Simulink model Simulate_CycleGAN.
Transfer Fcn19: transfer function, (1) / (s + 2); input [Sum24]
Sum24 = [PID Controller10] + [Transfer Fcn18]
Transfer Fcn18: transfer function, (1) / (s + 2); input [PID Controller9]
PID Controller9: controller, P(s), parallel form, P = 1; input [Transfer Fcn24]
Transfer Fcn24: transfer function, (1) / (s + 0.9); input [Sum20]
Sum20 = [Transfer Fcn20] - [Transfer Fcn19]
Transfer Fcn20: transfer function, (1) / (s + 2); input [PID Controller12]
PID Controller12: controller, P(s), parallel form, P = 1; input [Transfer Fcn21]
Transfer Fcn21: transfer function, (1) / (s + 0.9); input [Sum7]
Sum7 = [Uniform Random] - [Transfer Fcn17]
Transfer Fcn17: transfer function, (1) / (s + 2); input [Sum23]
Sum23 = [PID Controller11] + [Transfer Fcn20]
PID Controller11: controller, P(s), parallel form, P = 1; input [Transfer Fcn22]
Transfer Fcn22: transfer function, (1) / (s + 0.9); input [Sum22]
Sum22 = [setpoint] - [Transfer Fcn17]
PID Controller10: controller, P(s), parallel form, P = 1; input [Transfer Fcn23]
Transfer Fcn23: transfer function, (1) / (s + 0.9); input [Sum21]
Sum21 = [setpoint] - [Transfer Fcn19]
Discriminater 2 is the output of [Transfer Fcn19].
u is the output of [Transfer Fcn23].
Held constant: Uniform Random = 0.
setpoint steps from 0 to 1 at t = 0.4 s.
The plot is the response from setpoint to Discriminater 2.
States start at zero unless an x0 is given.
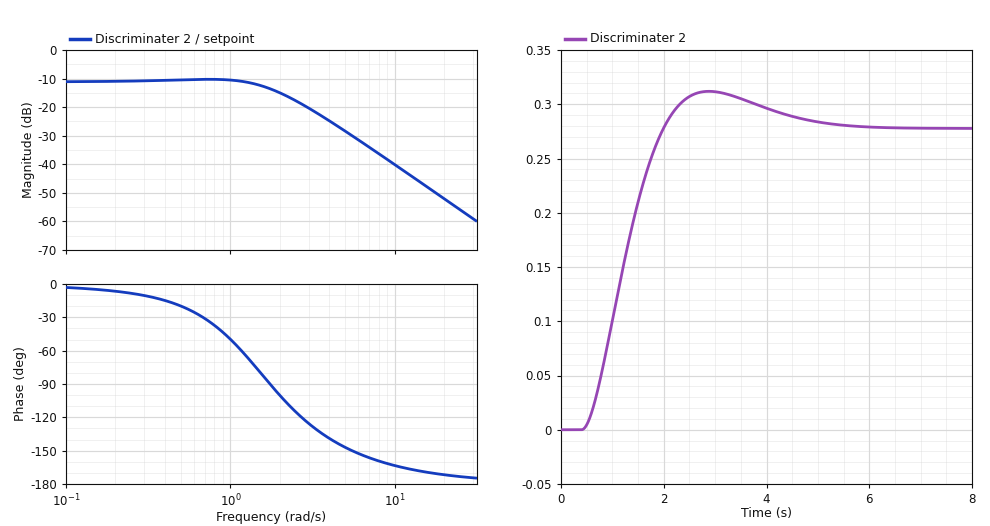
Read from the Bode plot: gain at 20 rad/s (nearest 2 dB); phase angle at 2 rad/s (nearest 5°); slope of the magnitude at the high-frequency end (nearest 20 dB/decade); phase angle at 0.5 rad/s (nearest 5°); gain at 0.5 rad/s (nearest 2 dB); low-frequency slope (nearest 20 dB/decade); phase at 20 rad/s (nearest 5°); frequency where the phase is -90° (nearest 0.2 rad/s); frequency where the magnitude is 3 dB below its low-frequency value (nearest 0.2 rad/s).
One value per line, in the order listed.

-52 dB
-100°
-40 dB/decade
-20°
-10 dB
0 dB/decade
-170°
1.8 rad/s
1.8 rad/s
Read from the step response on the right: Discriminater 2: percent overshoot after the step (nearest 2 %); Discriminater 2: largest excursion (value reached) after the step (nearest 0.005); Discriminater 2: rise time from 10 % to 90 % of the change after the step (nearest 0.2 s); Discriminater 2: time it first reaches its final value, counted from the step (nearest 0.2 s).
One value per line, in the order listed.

12 %
0.310
1.0 s
1.6 s
